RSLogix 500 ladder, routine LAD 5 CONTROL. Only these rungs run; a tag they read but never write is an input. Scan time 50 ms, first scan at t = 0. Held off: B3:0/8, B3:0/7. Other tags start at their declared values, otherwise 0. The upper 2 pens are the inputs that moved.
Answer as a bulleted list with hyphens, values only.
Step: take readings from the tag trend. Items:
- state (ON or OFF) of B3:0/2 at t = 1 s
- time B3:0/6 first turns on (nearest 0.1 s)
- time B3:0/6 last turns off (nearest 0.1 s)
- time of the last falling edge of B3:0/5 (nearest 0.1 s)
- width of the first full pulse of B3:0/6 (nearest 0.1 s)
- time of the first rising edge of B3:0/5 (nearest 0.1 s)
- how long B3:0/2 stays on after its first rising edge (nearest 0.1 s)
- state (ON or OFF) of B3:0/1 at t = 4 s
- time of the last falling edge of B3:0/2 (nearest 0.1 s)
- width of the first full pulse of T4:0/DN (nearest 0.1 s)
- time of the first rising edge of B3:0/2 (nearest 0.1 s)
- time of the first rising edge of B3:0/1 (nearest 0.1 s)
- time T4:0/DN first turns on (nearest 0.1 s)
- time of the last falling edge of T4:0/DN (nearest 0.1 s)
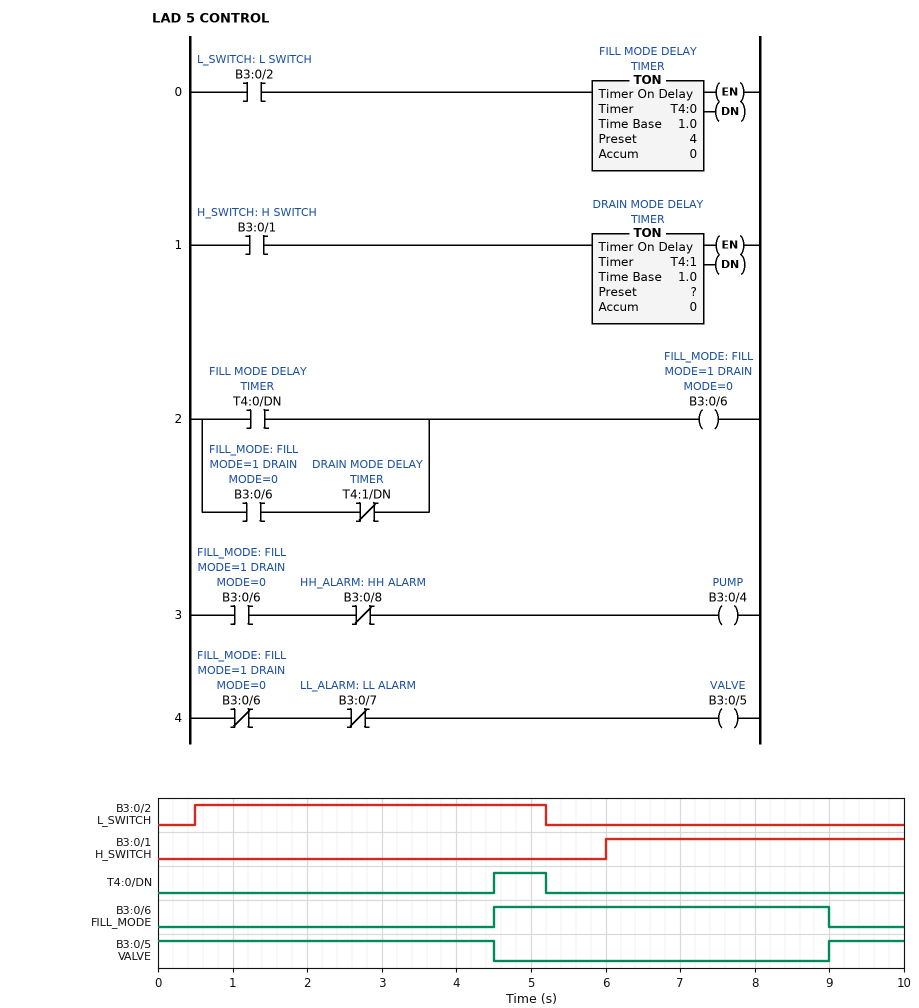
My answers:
- ON
- 4.5 s
- 9.0 s
- 4.5 s
- 4.5 s
- 9.0 s
- 4.7 s
- OFF
- 5.2 s
- 0.7 s
- 0.5 s
- 6.0 s
- 4.5 s
- 5.2 s
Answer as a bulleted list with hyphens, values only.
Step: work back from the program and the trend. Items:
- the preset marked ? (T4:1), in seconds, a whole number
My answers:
- 3 s
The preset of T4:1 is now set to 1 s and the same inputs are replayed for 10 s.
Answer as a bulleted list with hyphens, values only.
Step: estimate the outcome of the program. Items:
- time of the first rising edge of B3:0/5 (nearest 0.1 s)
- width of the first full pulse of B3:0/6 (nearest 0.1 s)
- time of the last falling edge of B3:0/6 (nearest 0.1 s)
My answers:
- 7.0 s
- 2.5 s
- 7.0 s
